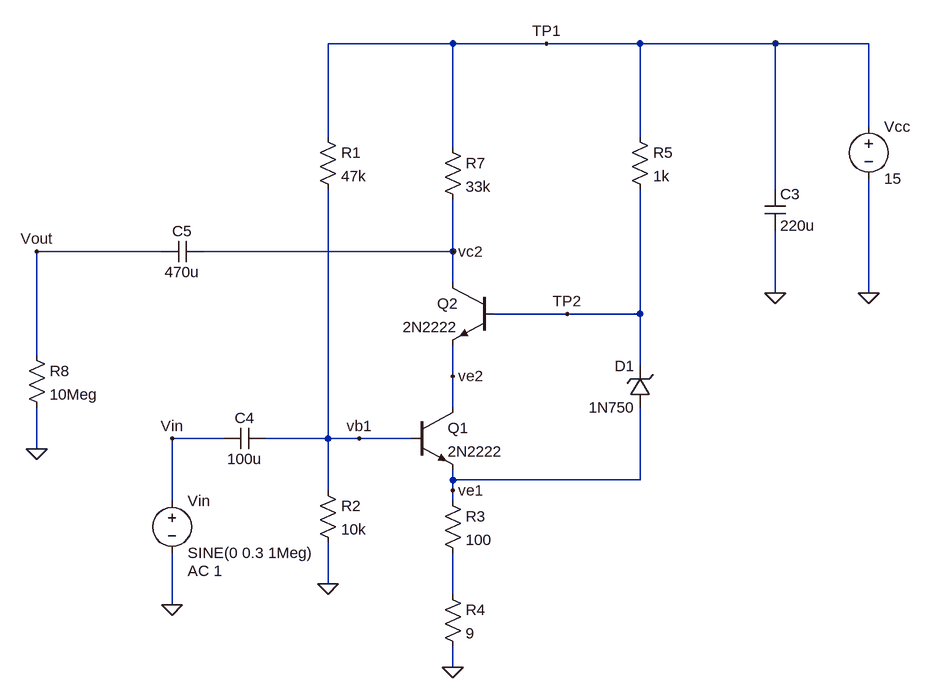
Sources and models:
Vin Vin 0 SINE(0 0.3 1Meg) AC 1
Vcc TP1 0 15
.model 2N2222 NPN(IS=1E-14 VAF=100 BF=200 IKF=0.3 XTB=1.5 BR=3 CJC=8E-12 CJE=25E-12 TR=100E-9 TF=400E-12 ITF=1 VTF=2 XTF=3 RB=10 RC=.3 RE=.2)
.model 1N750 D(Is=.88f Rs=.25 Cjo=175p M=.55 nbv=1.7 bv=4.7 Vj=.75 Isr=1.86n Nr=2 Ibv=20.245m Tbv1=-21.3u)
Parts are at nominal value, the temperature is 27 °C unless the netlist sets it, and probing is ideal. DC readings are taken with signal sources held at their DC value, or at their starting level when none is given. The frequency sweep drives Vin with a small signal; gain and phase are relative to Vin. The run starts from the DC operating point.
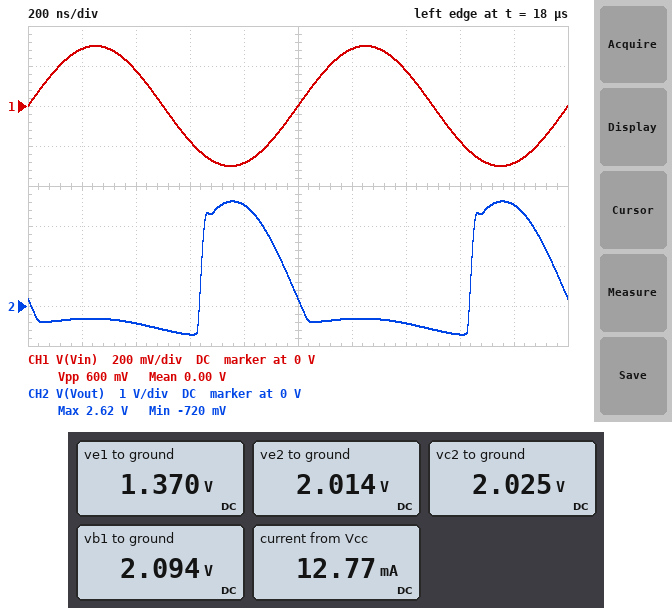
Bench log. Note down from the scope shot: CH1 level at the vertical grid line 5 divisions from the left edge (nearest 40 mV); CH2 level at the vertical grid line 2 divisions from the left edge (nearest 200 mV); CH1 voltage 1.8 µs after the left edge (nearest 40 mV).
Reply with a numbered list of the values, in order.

1. 0 V
2. -400 mV
3. -280 mV
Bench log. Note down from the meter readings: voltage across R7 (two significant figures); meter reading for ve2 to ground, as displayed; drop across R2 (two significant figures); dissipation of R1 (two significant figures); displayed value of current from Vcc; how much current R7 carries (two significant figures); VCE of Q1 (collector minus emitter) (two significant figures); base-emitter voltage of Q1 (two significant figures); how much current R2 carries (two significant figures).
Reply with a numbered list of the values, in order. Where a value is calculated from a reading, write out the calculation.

1. 15 V - 2.025 V = 13 V
2. 2.014 V
3. 2.094 V = 2.1 V
4. (15 V - 2.094 V)^2 / 47 kΩ = 3.5 mW
5. 12.77 mA
6. (15 V - 2.025 V) / 33 kΩ = 390 µA
7. 2.014 V - 1.37 V = 640 mV
8. 2.094 V - 1.37 V = 720 mV
9. (2.094 V) / 10 kΩ = 210 µA
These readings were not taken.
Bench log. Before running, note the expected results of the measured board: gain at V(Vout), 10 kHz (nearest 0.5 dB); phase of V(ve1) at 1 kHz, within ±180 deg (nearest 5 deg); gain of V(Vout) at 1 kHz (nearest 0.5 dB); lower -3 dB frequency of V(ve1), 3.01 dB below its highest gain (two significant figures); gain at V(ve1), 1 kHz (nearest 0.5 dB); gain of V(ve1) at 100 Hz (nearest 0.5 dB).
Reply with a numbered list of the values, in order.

1. 19.0 dB
2. 0 deg
3. 19.0 dB
4. 280 mHz
5. 0 dB
6. 0 dB
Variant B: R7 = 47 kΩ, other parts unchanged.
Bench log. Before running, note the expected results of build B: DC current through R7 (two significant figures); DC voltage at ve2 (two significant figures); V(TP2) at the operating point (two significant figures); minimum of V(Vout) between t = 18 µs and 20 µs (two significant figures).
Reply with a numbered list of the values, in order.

1. 280 µA
2. 1.9 V
3. 2.8 V
4. -620 mV
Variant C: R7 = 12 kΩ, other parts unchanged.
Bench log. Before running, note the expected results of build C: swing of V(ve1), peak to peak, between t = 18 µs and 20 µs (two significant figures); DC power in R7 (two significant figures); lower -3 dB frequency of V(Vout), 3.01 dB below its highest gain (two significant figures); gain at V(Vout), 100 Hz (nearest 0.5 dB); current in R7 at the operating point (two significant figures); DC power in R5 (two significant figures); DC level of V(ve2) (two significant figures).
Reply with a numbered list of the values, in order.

1. 550 mV
2. 13 mW
3. 290 mHz
4. 18.5 dB
5. 1.0 mA
6. 130 mW
7. 2.6 V
